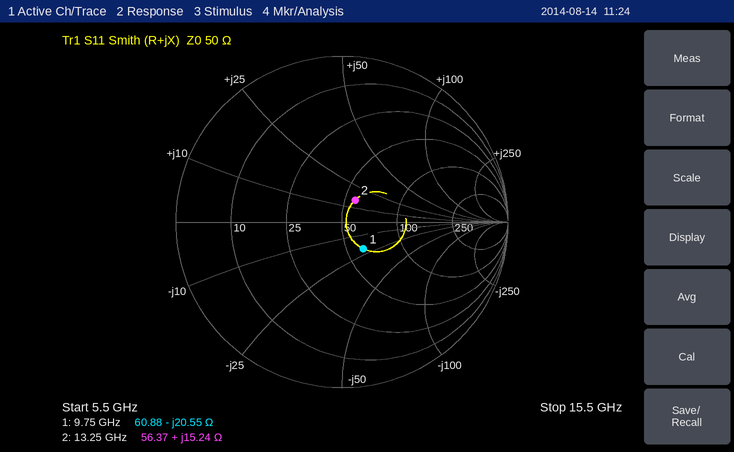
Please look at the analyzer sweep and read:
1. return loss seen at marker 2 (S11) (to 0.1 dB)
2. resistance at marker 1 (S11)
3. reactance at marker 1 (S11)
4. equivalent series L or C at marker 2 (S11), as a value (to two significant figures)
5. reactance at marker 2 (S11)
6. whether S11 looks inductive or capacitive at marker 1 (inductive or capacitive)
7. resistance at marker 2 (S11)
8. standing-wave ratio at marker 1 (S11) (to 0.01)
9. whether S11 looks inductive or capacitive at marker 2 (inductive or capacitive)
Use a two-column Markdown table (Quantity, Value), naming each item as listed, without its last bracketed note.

| Quantity | Value |
|---|---|
| return loss seen at marker 2 (S11) | 16.3 dB |
| resistance at marker 1 | 60.88 Ω |
| reactance at marker 1 | -20.55 Ω |
| equivalent series L or C at marker 2 (S11), as a value | 180 pH |
| reactance at marker 2 | +15.24 Ω |
| whether S11 looks inductive or capacitive at marker 1 | capacitive |
| resistance at marker 2 | 56.37 Ω |
| standing-wave ratio at marker 1 (S11) | 1.52 |
| whether S11 looks inductive or capacitive at marker 2 | inductive |
